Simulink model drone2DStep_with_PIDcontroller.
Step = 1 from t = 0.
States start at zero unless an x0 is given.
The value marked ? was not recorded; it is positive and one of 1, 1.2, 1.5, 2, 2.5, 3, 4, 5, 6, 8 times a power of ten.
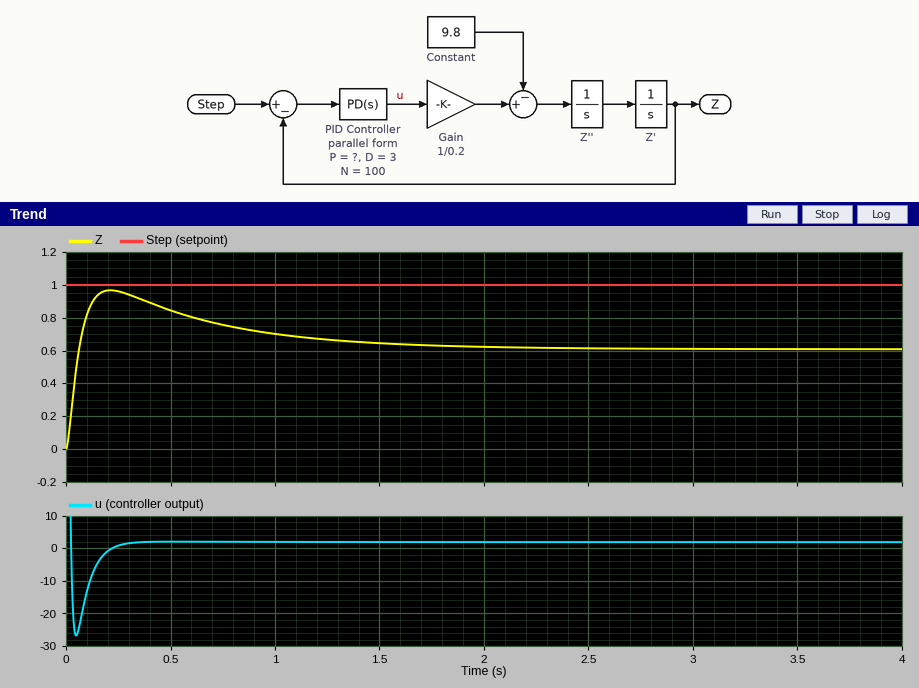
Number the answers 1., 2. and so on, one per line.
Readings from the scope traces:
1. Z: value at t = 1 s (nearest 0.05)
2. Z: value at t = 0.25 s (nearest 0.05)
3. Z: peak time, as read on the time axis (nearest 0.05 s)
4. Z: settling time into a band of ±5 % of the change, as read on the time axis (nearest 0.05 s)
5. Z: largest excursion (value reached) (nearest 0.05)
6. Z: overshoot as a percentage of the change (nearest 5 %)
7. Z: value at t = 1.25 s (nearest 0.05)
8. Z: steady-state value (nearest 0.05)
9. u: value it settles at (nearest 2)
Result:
1. 0.70
2. 0.95
3. 0.20 s
4. 1.60 s
5. 0.95
6. 60 %
7. 0.65
8. 0.60
9. 2
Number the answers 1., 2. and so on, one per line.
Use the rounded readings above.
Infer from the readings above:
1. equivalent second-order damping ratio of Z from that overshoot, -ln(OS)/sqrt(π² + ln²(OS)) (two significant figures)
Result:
1. 0.16
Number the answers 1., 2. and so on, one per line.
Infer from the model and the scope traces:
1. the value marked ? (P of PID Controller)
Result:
1. 5
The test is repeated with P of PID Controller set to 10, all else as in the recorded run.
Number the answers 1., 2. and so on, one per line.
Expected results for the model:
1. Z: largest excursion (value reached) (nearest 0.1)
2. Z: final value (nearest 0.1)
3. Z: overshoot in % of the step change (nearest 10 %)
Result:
1. 1.0
2. 0.8
3. 30 %
